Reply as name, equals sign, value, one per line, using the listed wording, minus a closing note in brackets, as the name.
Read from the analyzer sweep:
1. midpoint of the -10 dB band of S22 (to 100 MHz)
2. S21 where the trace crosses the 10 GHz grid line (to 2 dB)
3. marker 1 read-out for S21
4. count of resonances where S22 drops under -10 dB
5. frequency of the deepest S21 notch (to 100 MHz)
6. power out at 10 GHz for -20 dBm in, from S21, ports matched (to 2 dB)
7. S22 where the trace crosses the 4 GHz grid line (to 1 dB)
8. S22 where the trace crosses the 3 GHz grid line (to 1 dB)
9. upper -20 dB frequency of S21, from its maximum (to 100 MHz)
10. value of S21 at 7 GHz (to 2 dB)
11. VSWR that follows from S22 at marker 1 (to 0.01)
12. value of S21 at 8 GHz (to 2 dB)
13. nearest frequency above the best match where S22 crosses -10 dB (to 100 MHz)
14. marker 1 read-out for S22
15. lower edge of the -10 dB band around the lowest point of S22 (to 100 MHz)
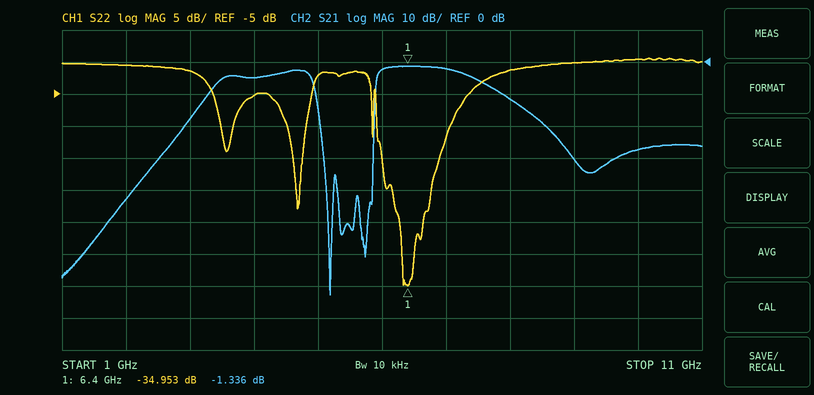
midpoint of the -10 dB band of S22 = 6.5 GHz
S21 where the trace crosses the 10 GHz grid line = -28 dB
marker 1 read-out for S21 = -1.336 dB
count of resonances where S22 drops under -10 dB = 4
frequency of the deepest S21 notch = 5.2 GHz
power out at 10 GHz for -20 dBm in, from S21, ports matched = -48 dBm
S22 where the trace crosses the 4 GHz grid line = -5 dB
S22 where the trace crosses the 3 GHz grid line = -1 dB
upper -20 dB frequency of S21, from its maximum = 8.6 GHz
value of S21 at 7 GHz = -2 dB
VSWR that follows from S22 at marker 1 = 1.04
value of S21 at 8 GHz = -12 dB
nearest frequency above the best match where S22 crosses -10 dB = 7.1 GHz
marker 1 read-out for S22 = -34.953 dB
lower edge of the -10 dB band around the lowest point of S22 = 5.9 GHz
